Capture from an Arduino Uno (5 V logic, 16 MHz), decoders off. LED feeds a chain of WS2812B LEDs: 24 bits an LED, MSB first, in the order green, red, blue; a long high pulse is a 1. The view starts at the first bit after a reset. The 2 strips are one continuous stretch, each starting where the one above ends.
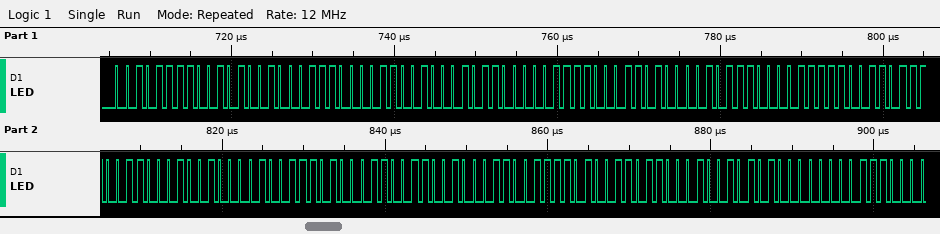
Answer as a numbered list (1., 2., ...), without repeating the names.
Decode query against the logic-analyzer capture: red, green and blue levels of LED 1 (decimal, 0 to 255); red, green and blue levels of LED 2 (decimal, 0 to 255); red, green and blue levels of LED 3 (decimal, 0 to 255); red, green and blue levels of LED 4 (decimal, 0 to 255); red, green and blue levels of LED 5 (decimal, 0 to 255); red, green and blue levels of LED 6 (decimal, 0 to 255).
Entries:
1. 41, 47, 28
2. 44, 50, 30
3. 46, 52, 31
4. 49, 55, 33
5. 51, 58, 35
6. 54, 61, 37
